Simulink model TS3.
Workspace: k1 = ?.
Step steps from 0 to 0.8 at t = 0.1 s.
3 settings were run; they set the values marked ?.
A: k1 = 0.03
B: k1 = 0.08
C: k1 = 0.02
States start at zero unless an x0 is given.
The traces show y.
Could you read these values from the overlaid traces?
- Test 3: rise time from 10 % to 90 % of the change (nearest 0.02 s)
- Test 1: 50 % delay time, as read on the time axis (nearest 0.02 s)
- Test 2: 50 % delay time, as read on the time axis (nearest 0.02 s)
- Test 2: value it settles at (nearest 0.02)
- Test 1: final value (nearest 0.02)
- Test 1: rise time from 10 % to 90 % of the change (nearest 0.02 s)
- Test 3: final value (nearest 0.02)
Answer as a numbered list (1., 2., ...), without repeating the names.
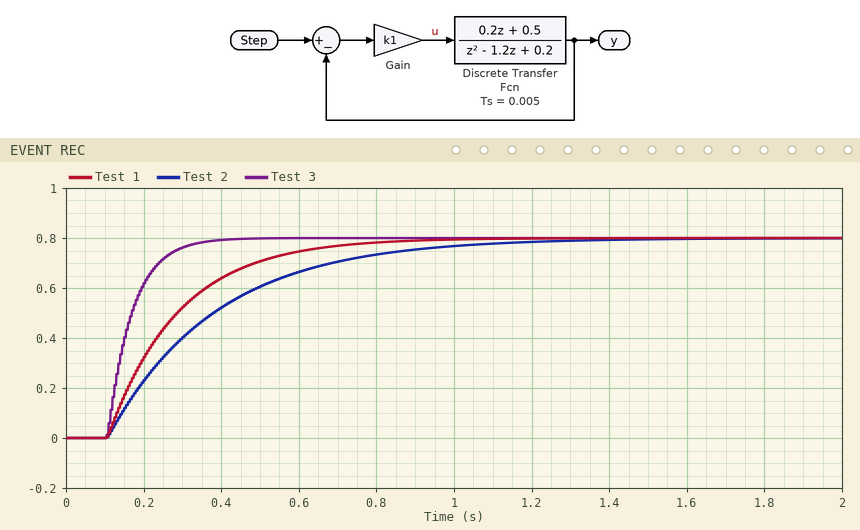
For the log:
1. 0.14 s
2. 0.24 s
3. 0.30 s
4. 0.80
5. 0.80
6. 0.40 s
7. 0.80
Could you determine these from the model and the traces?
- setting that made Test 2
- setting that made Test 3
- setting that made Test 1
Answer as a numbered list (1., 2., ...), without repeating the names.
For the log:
1. C
2. B
3. A
